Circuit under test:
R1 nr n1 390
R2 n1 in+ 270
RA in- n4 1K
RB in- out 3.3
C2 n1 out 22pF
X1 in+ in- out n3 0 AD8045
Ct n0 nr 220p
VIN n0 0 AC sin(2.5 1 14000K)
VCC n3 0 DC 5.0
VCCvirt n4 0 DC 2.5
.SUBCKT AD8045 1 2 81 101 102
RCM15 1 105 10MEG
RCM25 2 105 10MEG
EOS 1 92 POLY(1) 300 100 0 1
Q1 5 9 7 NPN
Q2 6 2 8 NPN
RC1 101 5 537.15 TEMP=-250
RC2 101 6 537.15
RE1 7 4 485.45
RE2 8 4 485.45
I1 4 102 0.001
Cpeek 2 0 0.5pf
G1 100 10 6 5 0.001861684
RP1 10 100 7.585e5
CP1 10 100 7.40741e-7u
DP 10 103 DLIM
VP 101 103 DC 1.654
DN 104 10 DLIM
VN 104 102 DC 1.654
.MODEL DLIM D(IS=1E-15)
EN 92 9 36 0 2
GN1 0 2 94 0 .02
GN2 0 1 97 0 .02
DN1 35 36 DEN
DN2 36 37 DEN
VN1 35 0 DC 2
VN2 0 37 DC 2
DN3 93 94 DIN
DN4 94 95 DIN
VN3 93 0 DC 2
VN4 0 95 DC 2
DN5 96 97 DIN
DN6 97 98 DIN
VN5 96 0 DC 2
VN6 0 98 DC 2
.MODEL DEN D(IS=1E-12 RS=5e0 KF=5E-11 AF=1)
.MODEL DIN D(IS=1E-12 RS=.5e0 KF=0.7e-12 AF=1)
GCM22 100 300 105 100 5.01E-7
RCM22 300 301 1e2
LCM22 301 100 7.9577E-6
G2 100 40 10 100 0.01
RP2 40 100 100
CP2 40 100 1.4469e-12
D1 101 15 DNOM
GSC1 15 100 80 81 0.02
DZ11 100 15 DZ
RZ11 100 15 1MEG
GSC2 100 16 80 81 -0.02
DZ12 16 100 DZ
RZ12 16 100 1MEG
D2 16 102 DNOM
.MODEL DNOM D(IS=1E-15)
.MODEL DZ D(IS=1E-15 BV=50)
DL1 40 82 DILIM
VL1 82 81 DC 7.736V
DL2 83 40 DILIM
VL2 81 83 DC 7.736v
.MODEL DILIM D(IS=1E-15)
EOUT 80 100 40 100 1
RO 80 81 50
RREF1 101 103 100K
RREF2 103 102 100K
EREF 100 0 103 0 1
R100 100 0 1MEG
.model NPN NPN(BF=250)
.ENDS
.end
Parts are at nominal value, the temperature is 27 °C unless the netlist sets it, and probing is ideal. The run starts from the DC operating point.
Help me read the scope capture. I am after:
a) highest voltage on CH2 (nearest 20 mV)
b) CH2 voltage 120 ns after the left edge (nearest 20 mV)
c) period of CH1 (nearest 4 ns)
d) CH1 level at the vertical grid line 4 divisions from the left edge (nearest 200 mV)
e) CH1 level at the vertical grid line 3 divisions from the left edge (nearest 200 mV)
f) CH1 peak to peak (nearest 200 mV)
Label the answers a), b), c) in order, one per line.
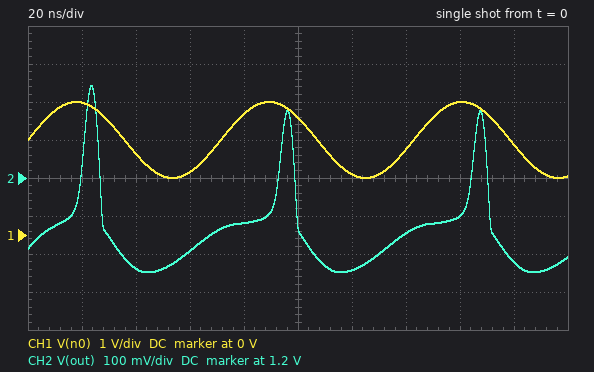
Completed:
a) 1.44 V
b) 960 mV
c) 72 ns
d) 3.2 V
e) 1.6 V
f) 2.0 V
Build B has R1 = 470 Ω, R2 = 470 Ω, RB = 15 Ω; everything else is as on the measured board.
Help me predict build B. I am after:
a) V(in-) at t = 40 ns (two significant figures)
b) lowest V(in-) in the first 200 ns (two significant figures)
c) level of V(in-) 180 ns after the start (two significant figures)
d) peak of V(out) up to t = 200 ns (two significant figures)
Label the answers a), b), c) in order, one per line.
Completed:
a) 990 mV
b) 980 mV
c) 1.0 V
d) 1.4 V
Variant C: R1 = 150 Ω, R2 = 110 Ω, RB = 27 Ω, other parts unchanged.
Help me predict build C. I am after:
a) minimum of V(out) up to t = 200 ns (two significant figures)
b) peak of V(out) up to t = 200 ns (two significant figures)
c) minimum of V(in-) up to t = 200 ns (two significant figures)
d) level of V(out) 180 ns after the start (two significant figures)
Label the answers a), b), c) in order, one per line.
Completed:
a) 940 mV
b) 1.5 V
c) 980 mV
d) 950 mV
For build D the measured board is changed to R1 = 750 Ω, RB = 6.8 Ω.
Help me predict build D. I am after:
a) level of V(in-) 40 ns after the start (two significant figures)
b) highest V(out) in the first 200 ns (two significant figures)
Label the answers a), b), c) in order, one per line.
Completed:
a) 1.0 V
b) 1.1 V
